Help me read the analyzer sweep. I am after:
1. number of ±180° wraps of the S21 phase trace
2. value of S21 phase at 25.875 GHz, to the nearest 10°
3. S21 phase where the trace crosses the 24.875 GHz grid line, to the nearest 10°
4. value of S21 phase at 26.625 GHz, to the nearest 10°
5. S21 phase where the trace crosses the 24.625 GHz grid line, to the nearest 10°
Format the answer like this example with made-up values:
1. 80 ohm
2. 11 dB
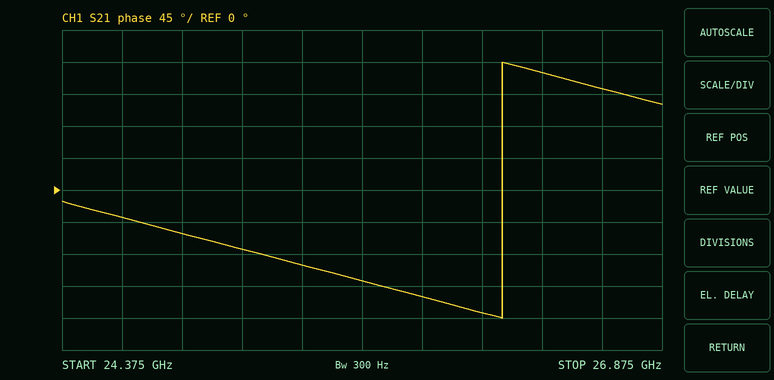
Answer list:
1. 1
2. -150°
3. -60°
4. 140°
5. -40°
